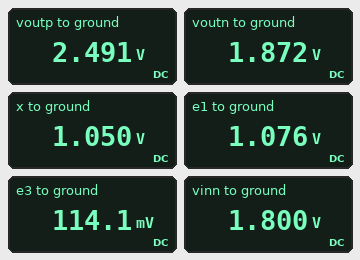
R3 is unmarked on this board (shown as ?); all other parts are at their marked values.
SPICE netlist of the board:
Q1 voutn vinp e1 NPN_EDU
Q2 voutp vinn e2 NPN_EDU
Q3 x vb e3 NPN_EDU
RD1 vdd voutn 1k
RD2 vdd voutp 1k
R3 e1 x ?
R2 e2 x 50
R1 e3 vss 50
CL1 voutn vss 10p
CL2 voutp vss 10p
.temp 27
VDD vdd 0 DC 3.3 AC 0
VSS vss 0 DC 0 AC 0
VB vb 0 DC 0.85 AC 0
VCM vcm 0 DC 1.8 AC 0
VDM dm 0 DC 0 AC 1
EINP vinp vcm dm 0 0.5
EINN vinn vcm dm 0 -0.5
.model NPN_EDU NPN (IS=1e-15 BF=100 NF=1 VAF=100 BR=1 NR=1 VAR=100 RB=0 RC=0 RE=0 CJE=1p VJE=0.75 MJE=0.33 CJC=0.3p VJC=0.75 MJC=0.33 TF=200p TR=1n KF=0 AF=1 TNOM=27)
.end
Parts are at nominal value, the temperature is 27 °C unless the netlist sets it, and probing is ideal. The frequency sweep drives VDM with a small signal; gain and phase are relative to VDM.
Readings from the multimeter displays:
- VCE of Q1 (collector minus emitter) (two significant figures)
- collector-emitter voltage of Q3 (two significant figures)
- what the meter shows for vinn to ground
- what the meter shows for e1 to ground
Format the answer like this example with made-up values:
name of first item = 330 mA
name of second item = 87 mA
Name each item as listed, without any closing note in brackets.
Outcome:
VCE of Q1 (collector minus emitter) = 800 mV
collector-emitter voltage of Q3 = 940 mV
what the meter shows for vinn to ground = 1.800 V
what the meter shows for e1 to ground = 1.076 V
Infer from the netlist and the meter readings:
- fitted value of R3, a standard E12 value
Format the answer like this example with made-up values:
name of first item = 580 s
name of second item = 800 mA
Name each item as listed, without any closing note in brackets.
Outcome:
fitted value of R3, a standard E12 value = 18 Ω
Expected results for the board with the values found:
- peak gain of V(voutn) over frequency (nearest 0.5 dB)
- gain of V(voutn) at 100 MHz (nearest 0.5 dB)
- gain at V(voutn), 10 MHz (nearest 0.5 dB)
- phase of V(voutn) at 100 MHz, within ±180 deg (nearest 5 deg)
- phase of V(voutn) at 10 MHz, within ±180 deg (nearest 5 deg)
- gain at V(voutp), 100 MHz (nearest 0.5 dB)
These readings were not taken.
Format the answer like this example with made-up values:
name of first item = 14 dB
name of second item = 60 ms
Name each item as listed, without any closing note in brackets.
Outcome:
peak gain of V(voutn) over frequency = 18.5 dB
gain of V(voutn) at 100 MHz = 2.0 dB
gain at V(voutn), 10 MHz = 17.0 dB
phase of V(voutn) at 100 MHz, within ±180 deg = 95 deg
phase of V(voutn) at 10 MHz, within ±180 deg = 145 deg
gain at V(voutp), 100 MHz = 2.0 dB
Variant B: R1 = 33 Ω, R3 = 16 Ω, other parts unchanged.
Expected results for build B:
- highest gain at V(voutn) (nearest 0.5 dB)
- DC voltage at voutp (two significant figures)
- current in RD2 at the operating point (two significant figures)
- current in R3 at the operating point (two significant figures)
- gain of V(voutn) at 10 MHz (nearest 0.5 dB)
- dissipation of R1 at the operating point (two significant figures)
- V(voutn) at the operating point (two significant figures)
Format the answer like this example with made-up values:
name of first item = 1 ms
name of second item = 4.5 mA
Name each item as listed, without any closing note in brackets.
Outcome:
highest gain at V(voutn) = 17.0 dB
DC voltage at voutp = 2.3 V
current in RD2 at the operating point = 1.0 mA
current in R3 at the operating point = 2.1 mA
gain of V(voutn) at 10 MHz = 16.0 dB
dissipation of R1 at the operating point = 340 µW
V(voutn) at the operating point = 1.2 V
